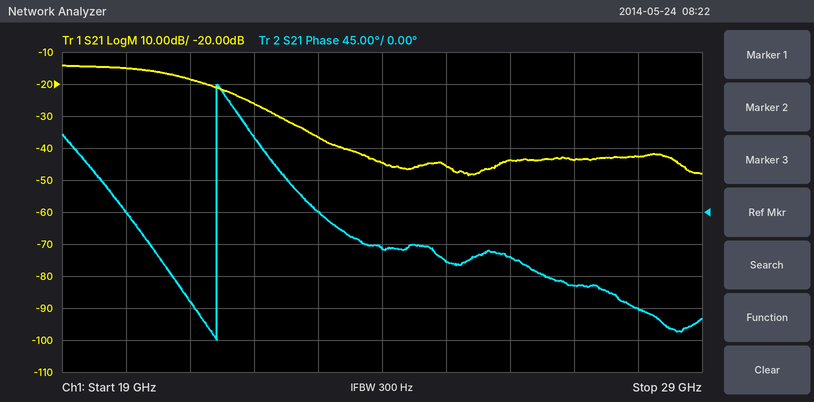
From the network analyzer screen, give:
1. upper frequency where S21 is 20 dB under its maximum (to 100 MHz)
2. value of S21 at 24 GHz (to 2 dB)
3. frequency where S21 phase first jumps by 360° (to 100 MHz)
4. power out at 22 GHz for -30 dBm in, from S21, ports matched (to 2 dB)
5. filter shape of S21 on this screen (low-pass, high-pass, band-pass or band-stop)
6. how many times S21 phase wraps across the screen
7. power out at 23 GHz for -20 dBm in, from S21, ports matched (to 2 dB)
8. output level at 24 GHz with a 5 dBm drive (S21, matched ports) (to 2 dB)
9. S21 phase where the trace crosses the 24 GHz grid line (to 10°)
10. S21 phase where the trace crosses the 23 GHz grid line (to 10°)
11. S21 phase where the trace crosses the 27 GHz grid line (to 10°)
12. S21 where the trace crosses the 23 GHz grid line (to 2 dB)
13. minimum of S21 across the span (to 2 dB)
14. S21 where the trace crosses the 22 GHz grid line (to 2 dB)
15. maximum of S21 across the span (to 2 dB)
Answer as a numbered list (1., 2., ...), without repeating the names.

1. 22.8 GHz
2. -44 dB
3. 21.4 GHz
4. -56 dBm
5. low-pass
6. 1
7. -56 dBm
8. -40 dBm
9. -50°
10. 0°
11. -100°
12. -36 dB
13. -48 dB
14. -26 dB
15. -14 dB
